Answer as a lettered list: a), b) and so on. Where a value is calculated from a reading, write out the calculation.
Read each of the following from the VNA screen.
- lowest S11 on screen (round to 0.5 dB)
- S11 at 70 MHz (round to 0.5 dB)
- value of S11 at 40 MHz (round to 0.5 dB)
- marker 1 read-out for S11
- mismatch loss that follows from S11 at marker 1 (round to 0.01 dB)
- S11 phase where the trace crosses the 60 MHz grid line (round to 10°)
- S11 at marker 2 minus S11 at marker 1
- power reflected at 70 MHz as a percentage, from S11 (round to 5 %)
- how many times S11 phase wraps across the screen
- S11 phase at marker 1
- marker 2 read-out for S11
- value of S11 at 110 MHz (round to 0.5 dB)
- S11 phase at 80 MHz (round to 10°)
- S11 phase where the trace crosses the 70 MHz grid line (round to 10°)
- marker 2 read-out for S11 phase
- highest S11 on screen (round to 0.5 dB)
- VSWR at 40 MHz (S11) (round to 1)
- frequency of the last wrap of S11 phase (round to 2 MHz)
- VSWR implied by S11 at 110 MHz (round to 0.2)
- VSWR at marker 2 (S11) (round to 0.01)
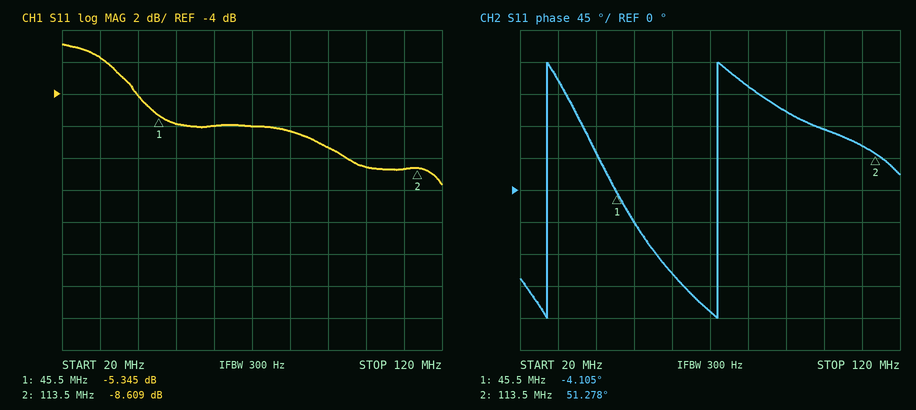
a) -9.5 dB
b) -6.0 dB
c) -4.0 dB
d) -5.345 dB
e) −10 log10(1 − 10^(-5.345/10)) ≈ 1.50 dB
f) -120°
g) -8.609 − (-5.345) = -3.264 dB
h) 10^(-6/10) ≈ 25 %
i) 2
j) -4.105°
k) -8.609 dB
l) -8.5 dB
m) 150°
n) -170°
o) 51.278°
p) -1.0 dB
q) |Γ| = 10^(-4/20) = 0.6310; VSWR = (1 + 0.6310)/(1 − 0.6310) ≈ 4
r) 72 MHz
s) |Γ| = 10^(-8.5/20) = 0.3758; VSWR = (1 + 0.3758)/(1 − 0.3758) ≈ 2.2
t) (1 + 0.3712)/(1 − 0.3712) ≈ 2.18
